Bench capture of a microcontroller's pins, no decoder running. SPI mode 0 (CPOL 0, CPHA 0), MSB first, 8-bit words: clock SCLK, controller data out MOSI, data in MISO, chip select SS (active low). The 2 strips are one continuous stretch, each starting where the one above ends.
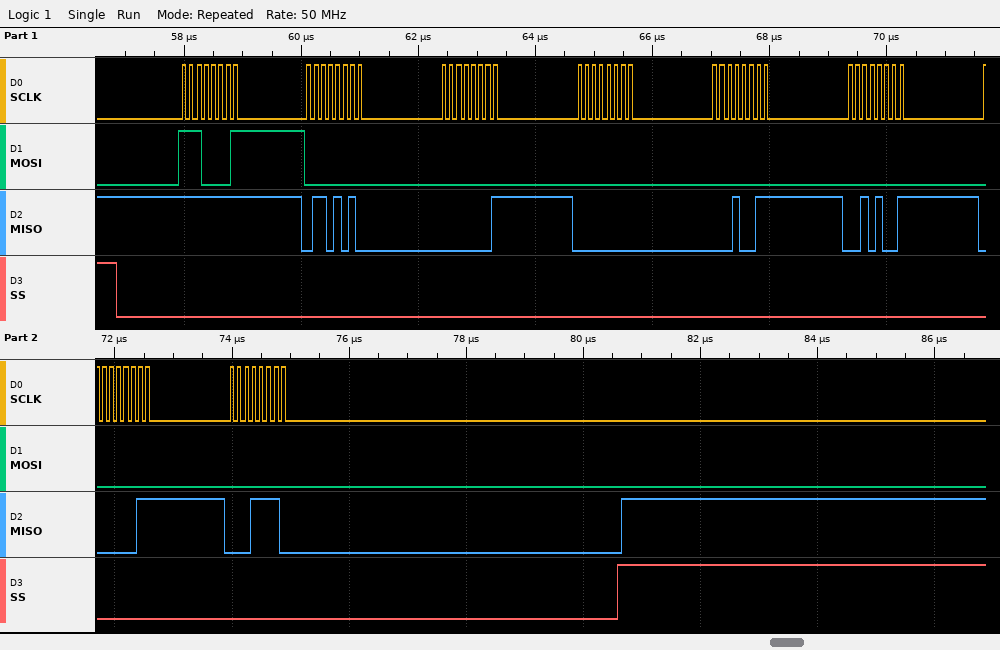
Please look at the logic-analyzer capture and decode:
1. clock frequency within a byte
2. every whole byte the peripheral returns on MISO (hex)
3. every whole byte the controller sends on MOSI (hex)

8 MHz
FF 6A 01 00 13 29 03 1E
E1 00 00 00 00 00 00 00
